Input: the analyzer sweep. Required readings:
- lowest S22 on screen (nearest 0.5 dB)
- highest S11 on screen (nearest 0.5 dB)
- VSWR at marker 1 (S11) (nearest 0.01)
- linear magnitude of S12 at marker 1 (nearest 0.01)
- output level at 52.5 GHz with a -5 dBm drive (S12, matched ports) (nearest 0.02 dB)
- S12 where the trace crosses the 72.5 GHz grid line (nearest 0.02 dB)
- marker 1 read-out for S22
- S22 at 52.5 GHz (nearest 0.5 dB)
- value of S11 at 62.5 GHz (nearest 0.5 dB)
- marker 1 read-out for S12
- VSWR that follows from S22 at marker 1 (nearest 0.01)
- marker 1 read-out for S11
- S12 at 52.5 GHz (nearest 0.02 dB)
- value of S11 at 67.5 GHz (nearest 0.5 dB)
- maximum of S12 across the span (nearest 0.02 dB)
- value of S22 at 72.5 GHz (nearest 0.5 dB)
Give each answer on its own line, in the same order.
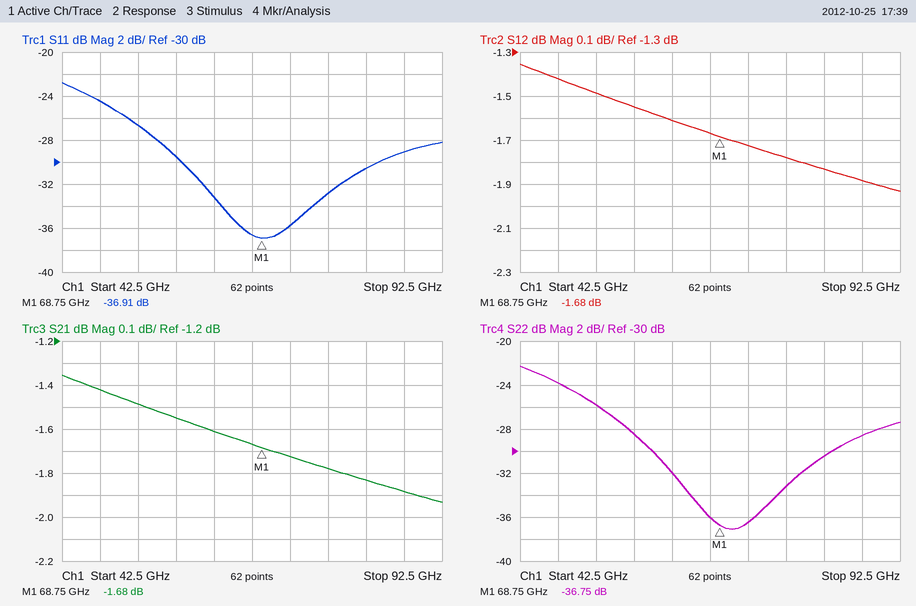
-37.0 dB
-23.0 dB
1.03
0.82
-6.48 dBm
-1.72 dB
-36.75 dB
-26.0 dB
-33.0 dB
-1.68 dB
1.03
-36.91 dB
-1.48 dB
-36.5 dB
-1.36 dB
-36.5 dB
